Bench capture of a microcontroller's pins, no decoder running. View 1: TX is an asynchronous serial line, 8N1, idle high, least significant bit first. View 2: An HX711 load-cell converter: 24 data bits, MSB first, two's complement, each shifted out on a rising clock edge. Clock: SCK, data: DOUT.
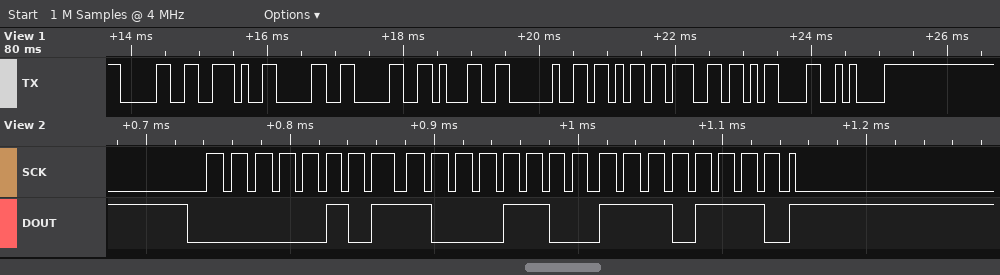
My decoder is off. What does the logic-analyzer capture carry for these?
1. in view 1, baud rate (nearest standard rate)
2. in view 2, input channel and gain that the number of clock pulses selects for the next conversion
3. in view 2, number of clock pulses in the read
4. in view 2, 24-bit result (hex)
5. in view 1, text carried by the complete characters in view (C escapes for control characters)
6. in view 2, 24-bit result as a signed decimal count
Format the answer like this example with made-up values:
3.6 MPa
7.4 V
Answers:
9600 baud
channel A, gain 128
25
0x058CEE
"0.001 kg\r\n"
363758
